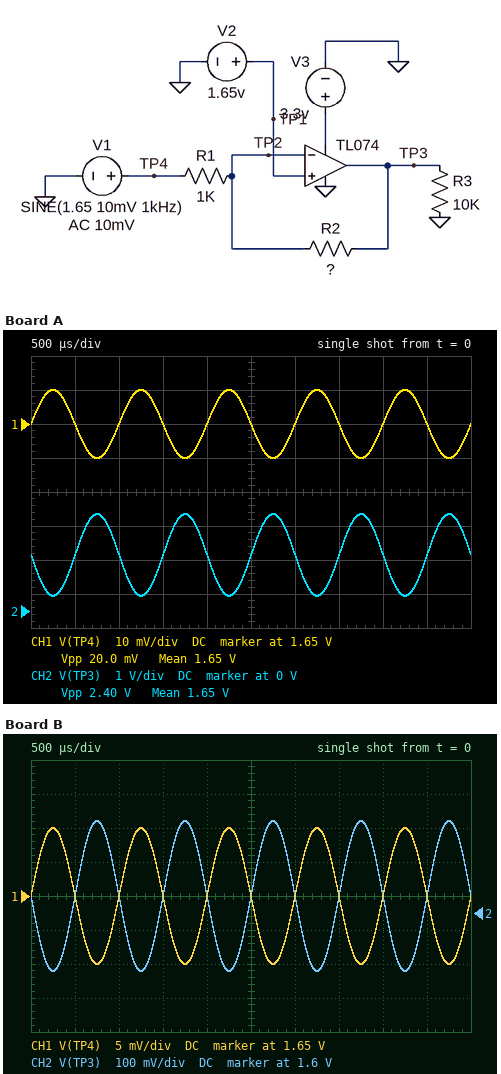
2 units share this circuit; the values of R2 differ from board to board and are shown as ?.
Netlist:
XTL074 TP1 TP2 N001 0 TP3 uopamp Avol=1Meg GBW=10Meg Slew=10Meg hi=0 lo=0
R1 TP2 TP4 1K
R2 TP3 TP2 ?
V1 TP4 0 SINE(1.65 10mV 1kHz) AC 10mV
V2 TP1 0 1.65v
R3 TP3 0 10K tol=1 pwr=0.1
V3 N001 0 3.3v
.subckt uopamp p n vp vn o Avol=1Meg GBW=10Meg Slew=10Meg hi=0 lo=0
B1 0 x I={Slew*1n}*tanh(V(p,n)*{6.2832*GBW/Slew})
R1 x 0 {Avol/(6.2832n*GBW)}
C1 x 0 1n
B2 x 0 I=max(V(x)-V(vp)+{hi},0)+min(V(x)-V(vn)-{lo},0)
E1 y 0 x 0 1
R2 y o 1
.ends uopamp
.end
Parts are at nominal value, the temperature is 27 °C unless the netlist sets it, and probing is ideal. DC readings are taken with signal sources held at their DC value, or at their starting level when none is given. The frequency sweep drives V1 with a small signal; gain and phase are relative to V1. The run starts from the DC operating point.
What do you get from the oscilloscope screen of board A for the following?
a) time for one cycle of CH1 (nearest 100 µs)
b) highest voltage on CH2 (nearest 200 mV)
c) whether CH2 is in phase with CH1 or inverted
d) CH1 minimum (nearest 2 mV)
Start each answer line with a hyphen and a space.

- 1.0 ms
- 2.8 V
- inverted
- 1.640 V
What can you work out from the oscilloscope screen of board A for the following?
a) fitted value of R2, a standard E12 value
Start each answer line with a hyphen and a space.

- 120 kΩ
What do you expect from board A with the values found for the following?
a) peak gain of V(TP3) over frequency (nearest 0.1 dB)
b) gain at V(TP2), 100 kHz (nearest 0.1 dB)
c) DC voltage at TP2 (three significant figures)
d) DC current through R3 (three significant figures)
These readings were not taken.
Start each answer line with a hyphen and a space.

- 41.6 dB
- -2.3 dB
- 1.65 V
- 165 µA
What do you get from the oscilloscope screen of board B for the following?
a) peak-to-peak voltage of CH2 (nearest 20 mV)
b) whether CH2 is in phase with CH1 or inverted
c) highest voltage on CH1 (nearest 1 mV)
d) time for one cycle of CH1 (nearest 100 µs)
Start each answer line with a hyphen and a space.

- 440 mV
- inverted
- 1.660 V
- 1.0 ms
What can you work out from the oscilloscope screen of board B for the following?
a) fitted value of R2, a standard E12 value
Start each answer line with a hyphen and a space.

- 22 kΩ
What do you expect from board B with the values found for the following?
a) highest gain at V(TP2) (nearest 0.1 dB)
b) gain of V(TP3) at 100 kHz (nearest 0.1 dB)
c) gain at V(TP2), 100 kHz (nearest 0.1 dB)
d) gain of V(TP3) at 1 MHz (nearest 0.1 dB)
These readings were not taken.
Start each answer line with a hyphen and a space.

- -0.4 dB
- 26.6 dB
- -13.4 dB
- 18.9 dB
